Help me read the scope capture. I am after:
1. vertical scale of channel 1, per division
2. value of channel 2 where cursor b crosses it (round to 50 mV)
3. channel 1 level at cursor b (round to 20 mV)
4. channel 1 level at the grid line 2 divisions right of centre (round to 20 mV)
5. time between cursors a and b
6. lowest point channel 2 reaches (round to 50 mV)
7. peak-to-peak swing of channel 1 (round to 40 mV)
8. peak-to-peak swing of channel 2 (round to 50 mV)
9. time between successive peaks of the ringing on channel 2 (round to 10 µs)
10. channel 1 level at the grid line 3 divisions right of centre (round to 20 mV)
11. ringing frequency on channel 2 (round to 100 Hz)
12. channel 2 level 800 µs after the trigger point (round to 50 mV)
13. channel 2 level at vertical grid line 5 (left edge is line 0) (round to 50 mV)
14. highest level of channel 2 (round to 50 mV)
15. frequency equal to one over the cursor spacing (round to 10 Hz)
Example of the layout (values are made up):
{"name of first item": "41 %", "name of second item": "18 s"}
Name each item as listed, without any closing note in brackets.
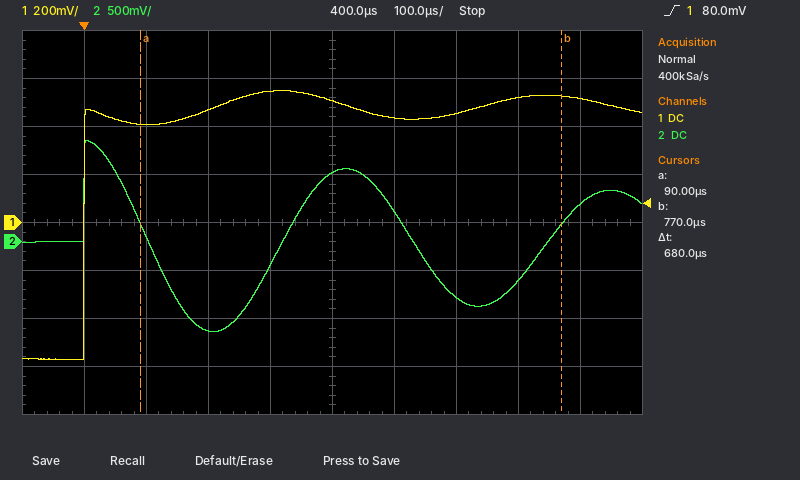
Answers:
{"vertical scale of channel 1, per division": "200 mV", "value of channel 2 where cursor b crosses it": "200 mV", "channel 1 level at cursor b": "520 mV", "channel 1 level at the grid line 2 divisions right of centre": "460 mV", "time between cursors a and b": "680 µs", "lowest point channel 2 reaches": "-950 mV", "peak-to-peak swing of channel 1": "1.12 V", "peak-to-peak swing of channel 2": "2.00 V", "time between successive peaks of the ringing on channel 2": "420 µs", "channel 1 level at the grid line 3 divisions right of centre": "520 mV", "ringing frequency on channel 2": "2.4 kHz", "channel 2 level 800 µs after the trigger point": "400 mV", "channel 2 level at vertical grid line 5 (left edge is line 0)": "700 mV", "highest level of channel 2": "1.05 V", "frequency equal to one over the cursor spacing": "1.47 kHz"}
